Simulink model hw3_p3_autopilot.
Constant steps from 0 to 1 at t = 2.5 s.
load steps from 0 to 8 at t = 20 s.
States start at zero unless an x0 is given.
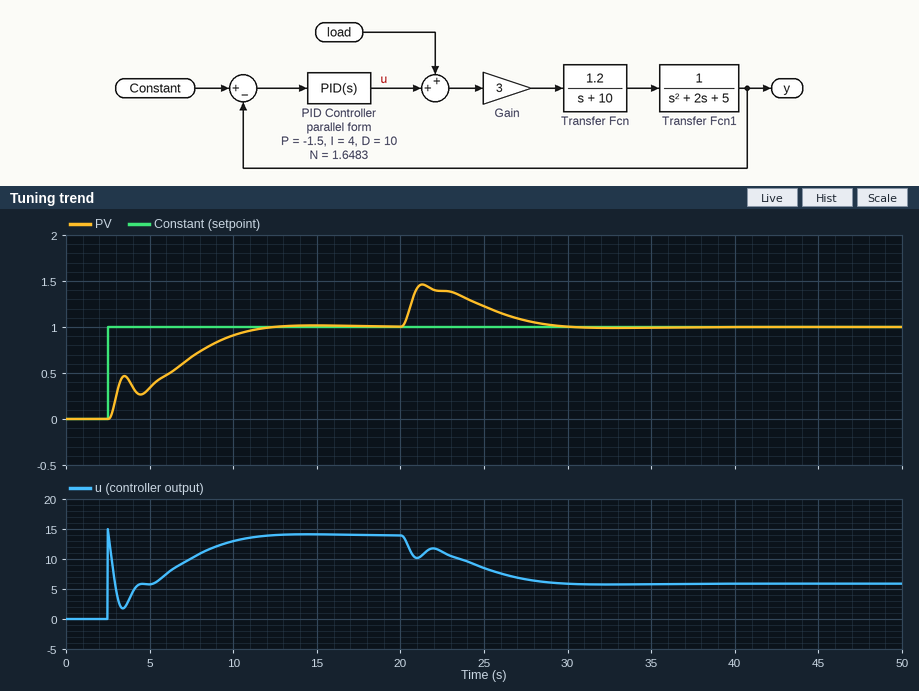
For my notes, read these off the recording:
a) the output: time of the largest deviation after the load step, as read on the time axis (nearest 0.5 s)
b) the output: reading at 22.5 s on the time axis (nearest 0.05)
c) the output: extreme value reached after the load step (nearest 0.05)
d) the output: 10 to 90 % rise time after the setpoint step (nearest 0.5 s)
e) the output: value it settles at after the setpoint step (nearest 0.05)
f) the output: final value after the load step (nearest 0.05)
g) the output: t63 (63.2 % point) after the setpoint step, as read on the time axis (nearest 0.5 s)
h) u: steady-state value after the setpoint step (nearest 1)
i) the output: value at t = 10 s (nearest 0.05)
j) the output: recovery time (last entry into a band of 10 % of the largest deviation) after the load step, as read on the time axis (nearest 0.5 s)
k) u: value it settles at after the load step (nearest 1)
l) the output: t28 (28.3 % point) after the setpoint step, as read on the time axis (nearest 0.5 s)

21.5 s
1.40
1.45
7.0 s
1.00
1.00
7.0 s
14
0.90
28.0 s
6
3.0 s
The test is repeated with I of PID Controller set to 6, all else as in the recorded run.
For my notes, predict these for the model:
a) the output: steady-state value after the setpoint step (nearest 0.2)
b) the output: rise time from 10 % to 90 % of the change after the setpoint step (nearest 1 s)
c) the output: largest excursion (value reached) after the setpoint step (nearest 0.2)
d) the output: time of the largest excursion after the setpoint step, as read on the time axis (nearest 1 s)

1.0
5 s
1.0
11 s
